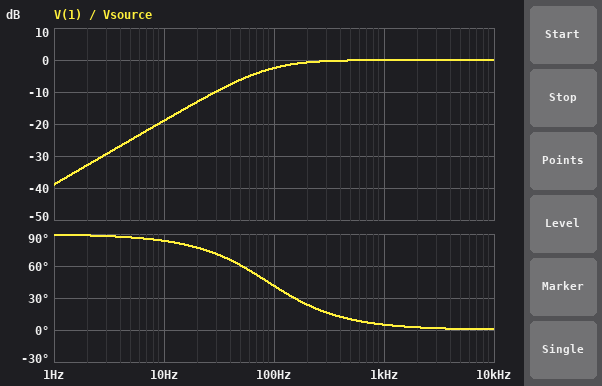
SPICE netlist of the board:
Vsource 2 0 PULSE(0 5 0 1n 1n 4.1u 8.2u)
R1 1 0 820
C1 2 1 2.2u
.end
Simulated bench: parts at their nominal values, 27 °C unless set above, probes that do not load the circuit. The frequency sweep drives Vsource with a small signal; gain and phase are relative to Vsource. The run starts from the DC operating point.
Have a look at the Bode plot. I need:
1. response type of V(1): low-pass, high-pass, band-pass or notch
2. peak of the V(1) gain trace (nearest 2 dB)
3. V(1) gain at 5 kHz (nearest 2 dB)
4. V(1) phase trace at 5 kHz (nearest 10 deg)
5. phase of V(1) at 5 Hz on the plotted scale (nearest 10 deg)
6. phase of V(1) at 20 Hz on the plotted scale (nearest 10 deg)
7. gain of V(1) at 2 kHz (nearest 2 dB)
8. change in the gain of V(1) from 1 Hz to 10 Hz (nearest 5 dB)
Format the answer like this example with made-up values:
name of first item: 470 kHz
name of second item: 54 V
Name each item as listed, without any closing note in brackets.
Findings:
response type of V(1): low-pass, high-pass, band-pass or notch: high-pass
peak of the V(1) gain trace: 0 dB
V(1) gain at 5 kHz: 0 dB
V(1) phase trace at 5 kHz: 0 deg
phase of V(1) at 5 Hz on the plotted scale: 90 deg
phase of V(1) at 20 Hz on the plotted scale: 80 deg
gain of V(1) at 2 kHz: 0 dB
change in the gain of V(1) from 1 Hz to 10 Hz: 20 dB
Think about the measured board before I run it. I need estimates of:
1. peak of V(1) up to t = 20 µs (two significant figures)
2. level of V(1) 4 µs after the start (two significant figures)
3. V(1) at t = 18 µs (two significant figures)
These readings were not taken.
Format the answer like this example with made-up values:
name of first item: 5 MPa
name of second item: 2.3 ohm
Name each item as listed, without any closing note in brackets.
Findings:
peak of V(1) up to t = 20 µs: 5.0 V
level of V(1) 4 µs after the start: 5.0 V
V(1) at t = 18 µs: 5.0 V
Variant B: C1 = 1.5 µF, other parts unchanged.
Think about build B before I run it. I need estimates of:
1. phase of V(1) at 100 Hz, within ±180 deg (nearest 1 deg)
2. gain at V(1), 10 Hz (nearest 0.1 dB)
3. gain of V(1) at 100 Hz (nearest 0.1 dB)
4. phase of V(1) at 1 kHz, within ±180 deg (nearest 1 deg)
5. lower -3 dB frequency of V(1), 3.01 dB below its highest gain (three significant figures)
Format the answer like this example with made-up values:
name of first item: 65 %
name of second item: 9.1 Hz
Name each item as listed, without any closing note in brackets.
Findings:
phase of V(1) at 100 Hz, within ±180 deg: 52 deg
gain at V(1), 10 Hz: -22.3 dB
gain of V(1) at 100 Hz: -4.3 dB
phase of V(1) at 1 kHz, within ±180 deg: 7 deg
lower -3 dB frequency of V(1), 3.01 dB below its highest gain: 129 Hz
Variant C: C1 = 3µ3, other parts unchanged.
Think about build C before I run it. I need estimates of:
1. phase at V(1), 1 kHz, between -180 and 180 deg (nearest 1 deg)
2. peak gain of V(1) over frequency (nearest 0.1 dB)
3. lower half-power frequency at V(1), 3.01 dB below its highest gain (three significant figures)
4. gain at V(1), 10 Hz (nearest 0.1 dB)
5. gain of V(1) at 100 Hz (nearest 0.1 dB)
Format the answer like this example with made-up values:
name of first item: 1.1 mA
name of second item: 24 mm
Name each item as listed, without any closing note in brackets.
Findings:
phase at V(1), 1 kHz, between -180 and 180 deg: 3 deg
peak gain of V(1) over frequency: 0 dB
lower half-power frequency at V(1), 3.01 dB below its highest gain: 58.8 Hz
gain at V(1), 10 Hz: -15.5 dB
gain of V(1) at 100 Hz: -1.3 dB
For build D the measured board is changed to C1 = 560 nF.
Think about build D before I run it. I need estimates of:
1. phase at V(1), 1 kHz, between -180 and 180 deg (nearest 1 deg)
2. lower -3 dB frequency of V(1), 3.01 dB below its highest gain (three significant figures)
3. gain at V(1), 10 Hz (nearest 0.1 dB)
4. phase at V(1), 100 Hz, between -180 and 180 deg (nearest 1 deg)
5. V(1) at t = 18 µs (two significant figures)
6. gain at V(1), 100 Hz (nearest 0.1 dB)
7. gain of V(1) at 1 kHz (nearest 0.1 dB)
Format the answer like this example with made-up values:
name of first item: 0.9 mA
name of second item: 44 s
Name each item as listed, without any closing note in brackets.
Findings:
phase at V(1), 1 kHz, between -180 and 180 deg: 19 deg
lower -3 dB frequency of V(1), 3.01 dB below its highest gain: 347 Hz
gain at V(1), 10 Hz: -30.8 dB
phase at V(1), 100 Hz, between -180 and 180 deg: 74 deg
V(1) at t = 18 µs: 4.9 V
gain at V(1), 100 Hz: -11.1 dB
gain of V(1) at 1 kHz: -0.5 dB
